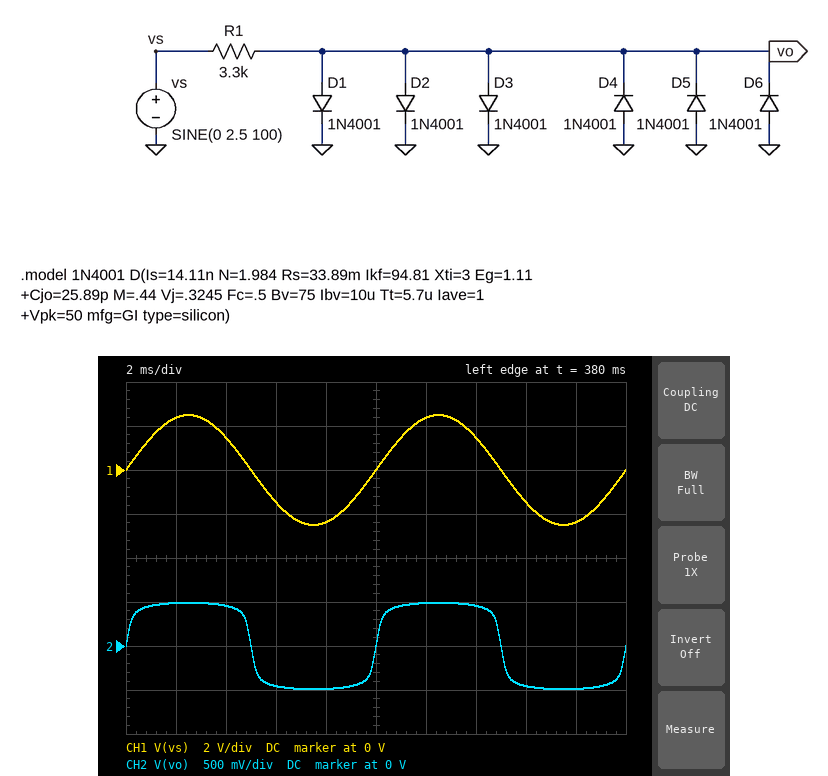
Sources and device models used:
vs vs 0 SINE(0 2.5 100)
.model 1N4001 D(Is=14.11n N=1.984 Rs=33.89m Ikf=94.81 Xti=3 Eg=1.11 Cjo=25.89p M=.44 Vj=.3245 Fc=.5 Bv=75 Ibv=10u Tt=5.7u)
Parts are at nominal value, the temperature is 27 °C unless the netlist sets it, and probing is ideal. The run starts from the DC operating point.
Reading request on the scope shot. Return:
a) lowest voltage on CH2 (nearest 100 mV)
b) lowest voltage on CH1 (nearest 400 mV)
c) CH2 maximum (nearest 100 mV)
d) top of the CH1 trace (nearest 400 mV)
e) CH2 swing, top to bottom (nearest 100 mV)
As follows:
-500 mV
-2.4 V
500 mV
2.4 V
1.0 V
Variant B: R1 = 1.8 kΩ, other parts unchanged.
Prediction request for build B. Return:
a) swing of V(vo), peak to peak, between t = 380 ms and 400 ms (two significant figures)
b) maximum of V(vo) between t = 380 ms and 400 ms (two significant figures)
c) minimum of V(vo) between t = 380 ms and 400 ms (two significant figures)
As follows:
1.0 V
520 mV
-520 mV
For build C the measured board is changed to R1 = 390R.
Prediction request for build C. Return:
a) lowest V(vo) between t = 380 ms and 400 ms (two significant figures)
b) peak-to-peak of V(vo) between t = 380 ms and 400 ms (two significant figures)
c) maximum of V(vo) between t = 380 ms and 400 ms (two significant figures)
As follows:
-600 mV
1.2 V
600 mV
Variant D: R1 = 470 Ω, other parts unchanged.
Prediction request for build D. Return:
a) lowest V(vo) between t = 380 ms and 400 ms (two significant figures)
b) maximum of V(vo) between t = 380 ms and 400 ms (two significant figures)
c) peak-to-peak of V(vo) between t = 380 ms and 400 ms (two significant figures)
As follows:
-590 mV
590 mV
1.2 V
